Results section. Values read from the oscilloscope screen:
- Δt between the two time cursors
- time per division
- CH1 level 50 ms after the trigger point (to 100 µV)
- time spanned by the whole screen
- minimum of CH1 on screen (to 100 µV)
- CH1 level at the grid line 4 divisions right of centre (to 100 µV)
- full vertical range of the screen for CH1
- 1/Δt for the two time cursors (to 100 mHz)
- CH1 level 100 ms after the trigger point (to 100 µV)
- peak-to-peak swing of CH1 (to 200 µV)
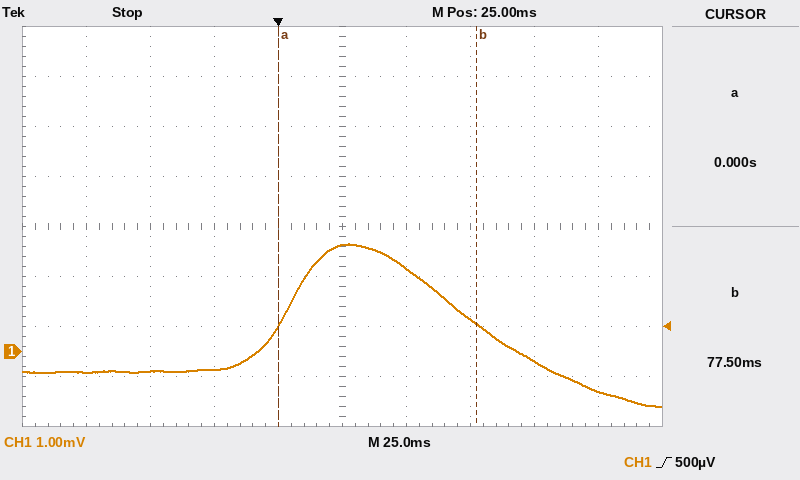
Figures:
77.5 ms
25 ms
1.7 mV
250 ms
-1.1 mV
-800 µV
8 mV
12.9 Hz
-200 µV
3.2 mV
